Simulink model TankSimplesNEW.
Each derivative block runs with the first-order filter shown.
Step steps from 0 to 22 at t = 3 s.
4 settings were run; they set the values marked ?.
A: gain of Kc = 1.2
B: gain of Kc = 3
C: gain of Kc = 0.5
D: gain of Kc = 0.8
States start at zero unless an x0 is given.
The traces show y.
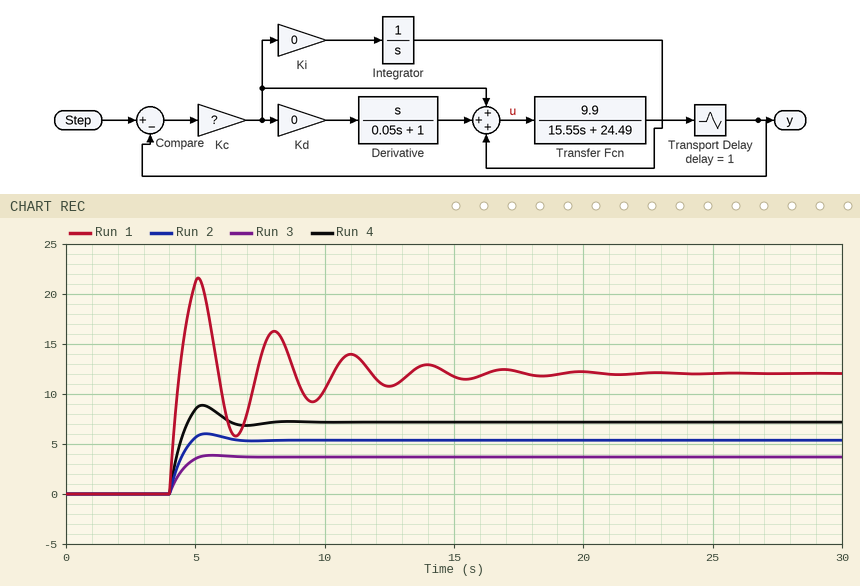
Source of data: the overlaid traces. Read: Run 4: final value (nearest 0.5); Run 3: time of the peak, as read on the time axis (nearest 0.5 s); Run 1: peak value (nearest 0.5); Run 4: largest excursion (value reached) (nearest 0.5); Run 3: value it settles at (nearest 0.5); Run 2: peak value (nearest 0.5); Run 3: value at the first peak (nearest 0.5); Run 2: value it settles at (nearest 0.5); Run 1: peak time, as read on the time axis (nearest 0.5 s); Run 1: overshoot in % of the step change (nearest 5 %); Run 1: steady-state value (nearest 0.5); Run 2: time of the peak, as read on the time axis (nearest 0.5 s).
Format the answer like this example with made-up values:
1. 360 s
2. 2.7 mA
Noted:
1. 7.0
2. 5.5 s
3. 21.5
4. 9.0
5. 3.5
6. 6.0
7. 4.0
8. 5.5
9. 5.0 s
10. 80 %
11. 12.0
12. 5.5 s
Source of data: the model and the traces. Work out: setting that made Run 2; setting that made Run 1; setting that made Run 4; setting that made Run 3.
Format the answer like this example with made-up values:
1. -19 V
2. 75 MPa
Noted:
1. D
2. B
3. A
4. C
